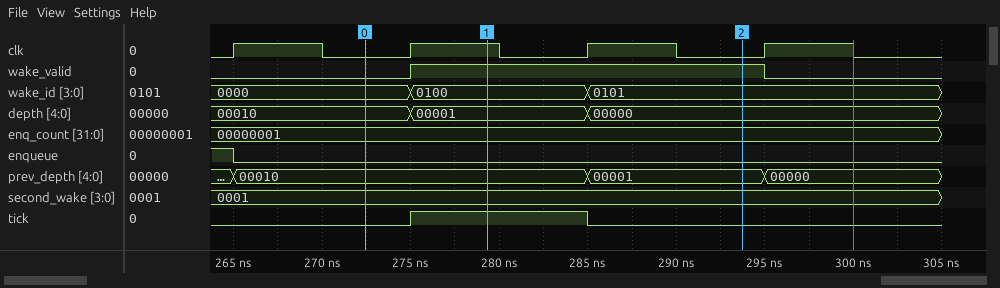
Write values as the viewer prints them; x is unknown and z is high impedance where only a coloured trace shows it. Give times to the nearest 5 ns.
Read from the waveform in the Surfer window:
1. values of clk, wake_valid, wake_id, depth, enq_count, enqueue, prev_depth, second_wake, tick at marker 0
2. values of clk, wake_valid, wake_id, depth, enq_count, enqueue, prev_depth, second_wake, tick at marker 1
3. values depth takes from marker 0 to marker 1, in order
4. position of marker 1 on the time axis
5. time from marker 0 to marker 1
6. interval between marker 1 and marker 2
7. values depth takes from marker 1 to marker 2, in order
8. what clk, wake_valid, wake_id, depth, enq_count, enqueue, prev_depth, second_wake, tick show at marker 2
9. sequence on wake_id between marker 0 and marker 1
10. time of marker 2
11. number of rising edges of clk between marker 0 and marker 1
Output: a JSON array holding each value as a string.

["clk=0, wake_valid=0, wake_id=0000, depth=00010, enq_count=00000001, enqueue=0, prev_depth=00010, second_wake=0001, tick=0", "clk=1, wake_valid=1, wake_id=0100, depth=00001, enq_count=00000001, enqueue=0, prev_depth=00010, second_wake=0001, tick=1", "00010, 00001", "280 ns", "5 ns", "15 ns", "00001, 00000", "clk=0, wake_valid=1, wake_id=0101, depth=00000, enq_count=00000001, enqueue=0, prev_depth=00001, second_wake=0001, tick=0", "0000, 0100", "295 ns", "1"]
